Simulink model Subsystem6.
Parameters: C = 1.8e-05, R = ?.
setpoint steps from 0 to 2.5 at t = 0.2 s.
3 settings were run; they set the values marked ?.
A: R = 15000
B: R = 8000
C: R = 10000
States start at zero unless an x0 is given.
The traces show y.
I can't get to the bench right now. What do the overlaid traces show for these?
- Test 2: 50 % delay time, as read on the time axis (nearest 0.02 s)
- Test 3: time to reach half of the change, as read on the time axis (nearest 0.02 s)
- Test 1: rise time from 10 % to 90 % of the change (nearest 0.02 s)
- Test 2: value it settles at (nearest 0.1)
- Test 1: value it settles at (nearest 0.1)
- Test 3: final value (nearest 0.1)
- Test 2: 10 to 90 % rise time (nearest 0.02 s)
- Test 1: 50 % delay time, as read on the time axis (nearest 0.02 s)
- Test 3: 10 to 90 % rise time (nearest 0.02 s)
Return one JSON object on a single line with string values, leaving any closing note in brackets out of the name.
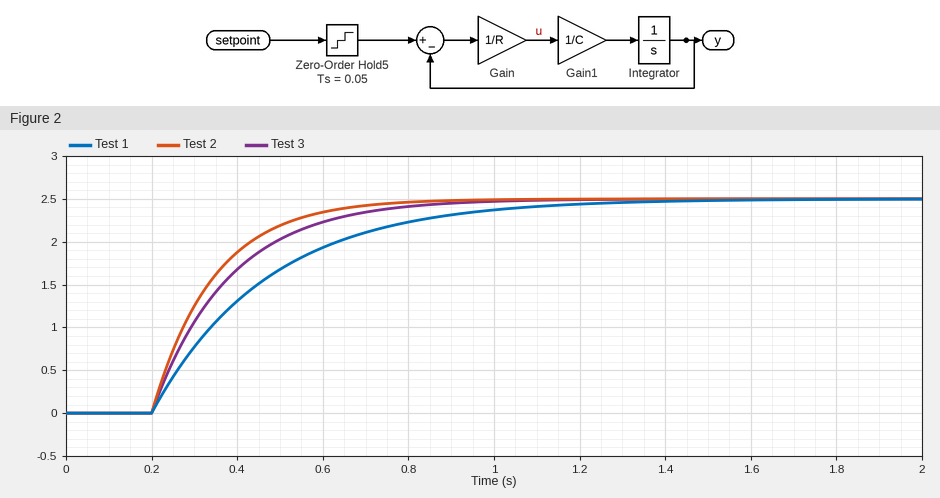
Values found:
{"Test 2: 50 % delay time, as read on the time axis": "0.30 s", "Test 3: time to reach half of the change, as read on the time axis": "0.32 s", "Test 1: rise time from 10 % to 90 % of the change": "0.60 s", "Test 2: value it settles at": "2.5", "Test 1: value it settles at": "2.5", "Test 3: final value": "2.5", "Test 2: 10 to 90 % rise time": "0.32 s", "Test 1: 50 % delay time, as read on the time axis": "0.38 s", "Test 3: 10 to 90 % rise time": "0.40 s"}
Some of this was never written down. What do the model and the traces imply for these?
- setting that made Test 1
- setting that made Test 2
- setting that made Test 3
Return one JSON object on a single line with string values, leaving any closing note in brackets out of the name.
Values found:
{"setting that made Test 1": "A", "setting that made Test 2": "B", "setting that made Test 3": "C"}
